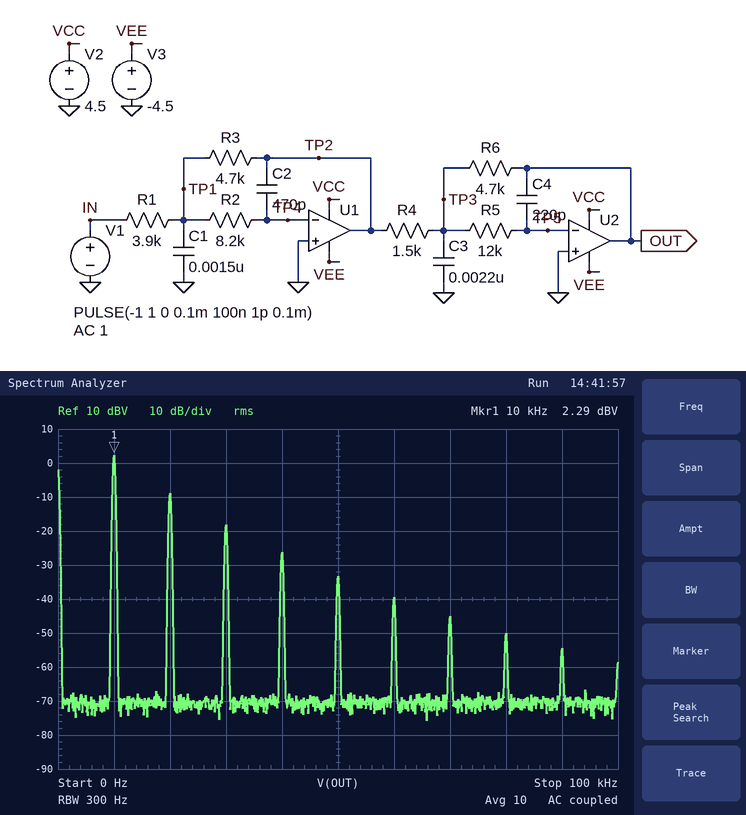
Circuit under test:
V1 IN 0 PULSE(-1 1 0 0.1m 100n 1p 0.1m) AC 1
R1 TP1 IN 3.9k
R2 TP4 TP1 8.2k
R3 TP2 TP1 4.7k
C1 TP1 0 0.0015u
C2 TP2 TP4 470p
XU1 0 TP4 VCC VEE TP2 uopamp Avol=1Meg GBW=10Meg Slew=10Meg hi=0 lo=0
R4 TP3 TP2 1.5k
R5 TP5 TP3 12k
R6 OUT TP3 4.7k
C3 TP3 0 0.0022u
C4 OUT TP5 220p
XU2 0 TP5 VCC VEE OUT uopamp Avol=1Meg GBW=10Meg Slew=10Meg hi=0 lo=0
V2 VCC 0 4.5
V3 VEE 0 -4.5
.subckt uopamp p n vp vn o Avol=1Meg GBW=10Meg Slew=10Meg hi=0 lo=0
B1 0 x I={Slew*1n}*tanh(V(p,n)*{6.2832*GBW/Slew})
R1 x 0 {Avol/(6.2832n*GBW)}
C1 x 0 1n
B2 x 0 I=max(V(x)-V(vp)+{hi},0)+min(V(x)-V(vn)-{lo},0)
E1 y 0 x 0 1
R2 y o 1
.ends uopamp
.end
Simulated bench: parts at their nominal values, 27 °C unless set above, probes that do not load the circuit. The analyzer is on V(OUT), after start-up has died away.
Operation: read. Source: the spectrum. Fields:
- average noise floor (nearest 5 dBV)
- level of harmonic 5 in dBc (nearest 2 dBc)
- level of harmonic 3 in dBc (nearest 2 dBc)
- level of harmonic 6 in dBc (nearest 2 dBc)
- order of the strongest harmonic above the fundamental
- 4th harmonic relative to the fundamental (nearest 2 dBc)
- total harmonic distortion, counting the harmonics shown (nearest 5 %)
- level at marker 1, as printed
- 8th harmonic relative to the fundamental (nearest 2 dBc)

-70 dBV
-36 dBc
-20 dBc
-42 dBc
2
-28 dBc
30 %
2.29 dBV
-52 dBc
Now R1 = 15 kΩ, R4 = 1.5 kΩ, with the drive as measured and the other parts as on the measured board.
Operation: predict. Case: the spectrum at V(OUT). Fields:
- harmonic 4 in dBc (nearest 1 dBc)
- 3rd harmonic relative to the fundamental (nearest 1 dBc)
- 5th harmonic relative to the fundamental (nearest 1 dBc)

-26 dBc
-18 dBc
-34 dBc
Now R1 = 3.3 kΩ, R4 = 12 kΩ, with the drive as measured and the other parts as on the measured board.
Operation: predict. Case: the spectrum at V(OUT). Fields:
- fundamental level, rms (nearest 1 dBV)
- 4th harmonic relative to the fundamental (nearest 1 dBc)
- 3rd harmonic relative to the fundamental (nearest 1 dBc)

-13 dBV
-24 dBc
-15 dBc
